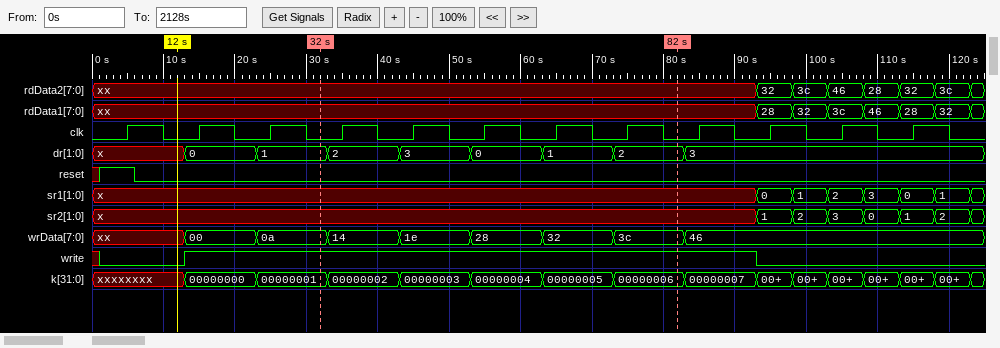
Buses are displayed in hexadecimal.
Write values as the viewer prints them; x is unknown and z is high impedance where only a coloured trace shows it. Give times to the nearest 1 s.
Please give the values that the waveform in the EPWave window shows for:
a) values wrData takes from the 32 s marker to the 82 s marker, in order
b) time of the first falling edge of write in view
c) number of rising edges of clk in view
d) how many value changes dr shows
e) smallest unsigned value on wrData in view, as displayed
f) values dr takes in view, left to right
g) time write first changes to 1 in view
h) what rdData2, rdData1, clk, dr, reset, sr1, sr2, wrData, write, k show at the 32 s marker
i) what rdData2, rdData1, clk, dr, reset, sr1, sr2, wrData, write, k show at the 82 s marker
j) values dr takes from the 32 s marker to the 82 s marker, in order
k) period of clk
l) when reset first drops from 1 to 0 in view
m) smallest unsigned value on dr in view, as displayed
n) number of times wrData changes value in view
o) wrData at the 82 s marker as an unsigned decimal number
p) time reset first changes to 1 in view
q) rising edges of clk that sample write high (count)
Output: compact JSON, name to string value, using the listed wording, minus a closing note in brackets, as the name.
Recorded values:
{"values wrData takes from the 32 s marker to the 82 s marker, in order": "0a, 14, 1e, 28, 32, 3c", "time of the first falling edge of write in view": "93 s", "number of rising edges of clk in view": "12", "how many value changes dr shows": "8", "smallest unsigned value on wrData in view, as displayed": "00", "values dr takes in view, left to right": "x, 0, 1, 2, 3, 0, 1, 2, 3", "time write first changes to 1 in view": "13 s", "what rdData2, rdData1, clk, dr, reset, sr1, sr2, wrData, write, k show at the 32 s marker": "rdData2=xx, rdData1=xx, clk=0, dr=1, reset=0, sr1=x, sr2=x, wrData=0a, write=1, k=00000001", "what rdData2, rdData1, clk, dr, reset, sr1, sr2, wrData, write, k show at the 82 s marker": "rdData2=xx, rdData1=xx, clk=0, dr=2, reset=0, sr1=x, sr2=x, wrData=3c, write=1, k=00000006", "values dr takes from the 32 s marker to the 82 s marker, in order": "1, 2, 3, 0, 1, 2", "period of clk": "10 s", "when reset first drops from 1 to 0 in view": "6 s", "smallest unsigned value on dr in view, as displayed": "0", "number of times wrData changes value in view": "8", "wrData at the 82 s marker as an unsigned decimal number": "60", "time reset first changes to 1 in view": "1 s", "rising edges of clk that sample write high": "8"}
